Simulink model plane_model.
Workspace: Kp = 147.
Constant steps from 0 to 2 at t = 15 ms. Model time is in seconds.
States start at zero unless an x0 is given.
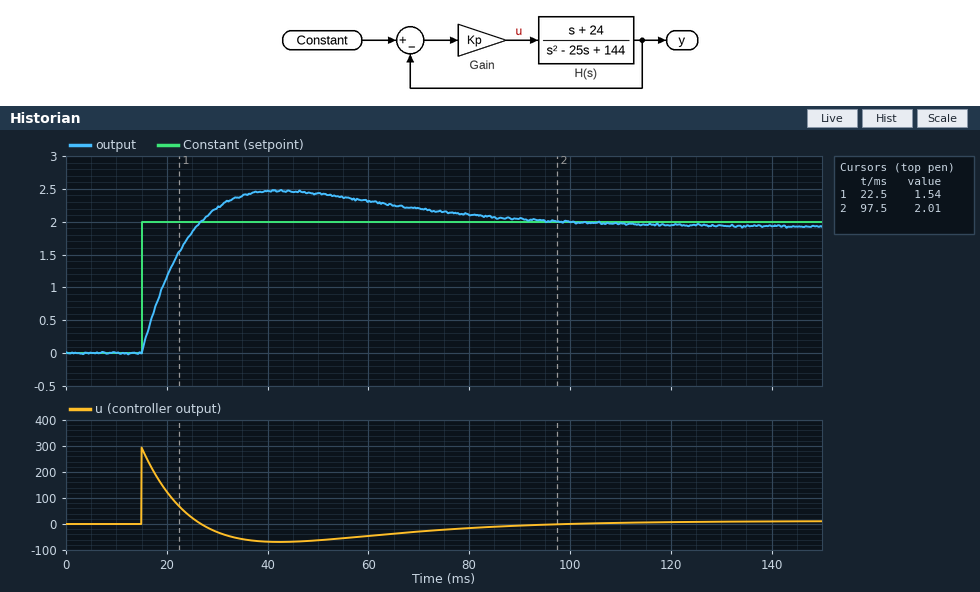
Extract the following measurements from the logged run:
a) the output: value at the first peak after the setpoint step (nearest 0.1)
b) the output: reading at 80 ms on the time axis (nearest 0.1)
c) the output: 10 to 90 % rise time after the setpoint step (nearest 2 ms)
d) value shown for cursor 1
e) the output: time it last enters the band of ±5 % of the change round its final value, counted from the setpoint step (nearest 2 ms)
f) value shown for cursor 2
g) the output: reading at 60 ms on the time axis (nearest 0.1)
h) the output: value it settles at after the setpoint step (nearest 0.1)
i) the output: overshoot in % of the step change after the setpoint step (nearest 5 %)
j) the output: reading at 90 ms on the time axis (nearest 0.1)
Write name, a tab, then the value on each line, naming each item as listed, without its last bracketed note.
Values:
the output: value at the first peak after the setpoint step	2.5
the output: reading at 80 ms on the time axis	2.1
the output: 10 to 90 % rise time after the setpoint step	8 ms
value shown for cursor 1	1.54
the output: time it last enters the band of ±5 % of the change round its final value, counted from the setpoint step	80 ms
value shown for cursor 2	2.01
the output: reading at 60 ms on the time axis	2.3
the output: value it settles at after the setpoint step	1.9
the output: overshoot in % of the step change after the setpoint step	30 %
the output: reading at 90 ms on the time axis	2.0
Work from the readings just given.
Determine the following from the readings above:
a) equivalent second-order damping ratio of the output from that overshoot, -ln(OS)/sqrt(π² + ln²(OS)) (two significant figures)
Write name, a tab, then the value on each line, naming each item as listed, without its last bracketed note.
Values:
equivalent second-order damping ratio of the output from that overshoot, -ln(OS)/sqrt(π² + ln²(OS))	0.36
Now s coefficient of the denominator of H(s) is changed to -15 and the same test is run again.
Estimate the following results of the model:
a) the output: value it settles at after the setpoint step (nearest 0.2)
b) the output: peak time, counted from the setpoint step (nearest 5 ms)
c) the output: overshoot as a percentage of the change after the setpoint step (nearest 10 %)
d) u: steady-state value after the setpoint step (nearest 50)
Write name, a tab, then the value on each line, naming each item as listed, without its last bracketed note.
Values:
the output: value it settles at after the setpoint step	2.0
the output: peak time, counted from the setpoint step	30 ms
the output: overshoot as a percentage of the change after the setpoint step	20 %
u: steady-state value after the setpoint step	0
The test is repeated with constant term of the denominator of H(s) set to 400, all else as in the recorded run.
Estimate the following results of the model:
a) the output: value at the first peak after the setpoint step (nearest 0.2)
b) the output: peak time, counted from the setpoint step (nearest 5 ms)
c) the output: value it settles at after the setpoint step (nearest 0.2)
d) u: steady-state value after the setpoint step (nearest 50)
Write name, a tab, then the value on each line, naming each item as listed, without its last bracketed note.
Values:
the output: value at the first peak after the setpoint step	2.4
the output: peak time, counted from the setpoint step	25 ms
the output: value it settles at after the setpoint step	1.8
u: steady-state value after the setpoint step	50
